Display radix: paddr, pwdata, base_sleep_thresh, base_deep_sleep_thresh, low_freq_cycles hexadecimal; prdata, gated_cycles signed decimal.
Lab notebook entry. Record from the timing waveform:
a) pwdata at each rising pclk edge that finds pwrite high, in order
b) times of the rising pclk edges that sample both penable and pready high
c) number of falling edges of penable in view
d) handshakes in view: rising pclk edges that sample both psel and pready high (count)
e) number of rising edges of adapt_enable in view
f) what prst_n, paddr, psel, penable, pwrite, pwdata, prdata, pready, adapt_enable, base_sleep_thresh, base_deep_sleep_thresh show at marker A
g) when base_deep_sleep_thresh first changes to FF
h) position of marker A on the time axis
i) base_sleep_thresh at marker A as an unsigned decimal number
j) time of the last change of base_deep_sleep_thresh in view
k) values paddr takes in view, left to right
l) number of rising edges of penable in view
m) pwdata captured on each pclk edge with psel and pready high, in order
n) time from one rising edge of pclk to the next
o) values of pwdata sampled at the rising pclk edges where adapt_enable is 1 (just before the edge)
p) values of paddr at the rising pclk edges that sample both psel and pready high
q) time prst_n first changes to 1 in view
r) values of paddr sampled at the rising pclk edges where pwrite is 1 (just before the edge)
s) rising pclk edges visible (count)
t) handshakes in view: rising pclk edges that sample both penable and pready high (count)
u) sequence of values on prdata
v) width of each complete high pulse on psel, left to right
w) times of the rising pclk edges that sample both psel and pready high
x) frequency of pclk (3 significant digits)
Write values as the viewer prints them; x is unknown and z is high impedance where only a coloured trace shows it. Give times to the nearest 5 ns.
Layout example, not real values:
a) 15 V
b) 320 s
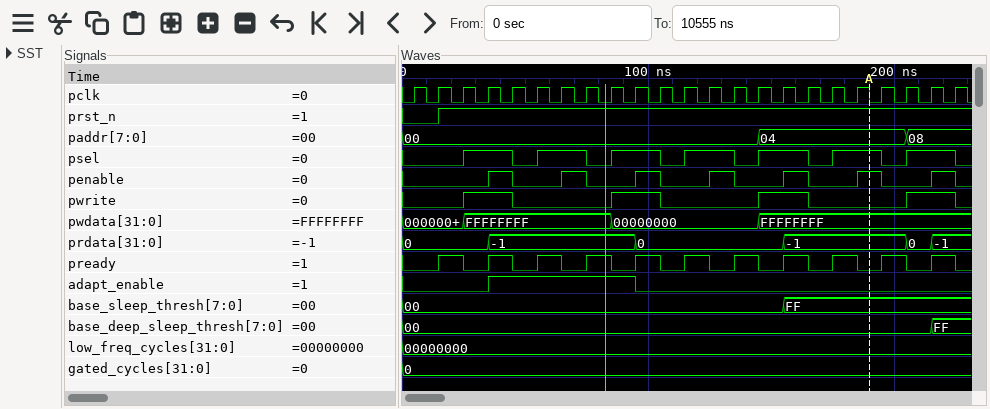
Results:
a) FFFFFFFF, FFFFFFFF, 00000000, 00000000, FFFFFFFF, FFFFFFFF, FFFFFFFF, FFFFFFFF
b) 45 ns, 105 ns, 165 ns, 225 ns
c) 7
d) 7
e) 1
f) prst_n=1, paddr=04, psel=1, penable=1, pwrite=0, pwdata=FFFFFFFF, prdata=-1, pready=0, adapt_enable=0, base_sleep_thresh=FF, base_deep_sleep_thresh=00
g) 215 ns
h) 190 ns
i) 255
j) 215 ns
k) 00, 04, 08
l) 7
m) FFFFFFFF, FFFFFFFF, 00000000, 00000000, FFFFFFFF, FFFFFFFF, FFFFFFFF
n) 10 ns
o) FFFFFFFF, FFFFFFFF, FFFFFFFF, FFFFFFFF, FFFFFFFF, 00000000
p) 00, 00, 00, 00, 04, 04, 08
q) 15 ns
r) 00, 00, 00, 00, 04, 04, 08, 08
s) 23
t) 4
u) 0, -1, 0, -1, 0, -1
v) 20 ns, 20 ns, 20 ns, 20 ns, 20 ns, 20 ns, 20 ns
w) 45 ns, 65 ns, 105 ns, 125 ns, 165 ns, 185 ns, 225 ns
x) 100 MHz
